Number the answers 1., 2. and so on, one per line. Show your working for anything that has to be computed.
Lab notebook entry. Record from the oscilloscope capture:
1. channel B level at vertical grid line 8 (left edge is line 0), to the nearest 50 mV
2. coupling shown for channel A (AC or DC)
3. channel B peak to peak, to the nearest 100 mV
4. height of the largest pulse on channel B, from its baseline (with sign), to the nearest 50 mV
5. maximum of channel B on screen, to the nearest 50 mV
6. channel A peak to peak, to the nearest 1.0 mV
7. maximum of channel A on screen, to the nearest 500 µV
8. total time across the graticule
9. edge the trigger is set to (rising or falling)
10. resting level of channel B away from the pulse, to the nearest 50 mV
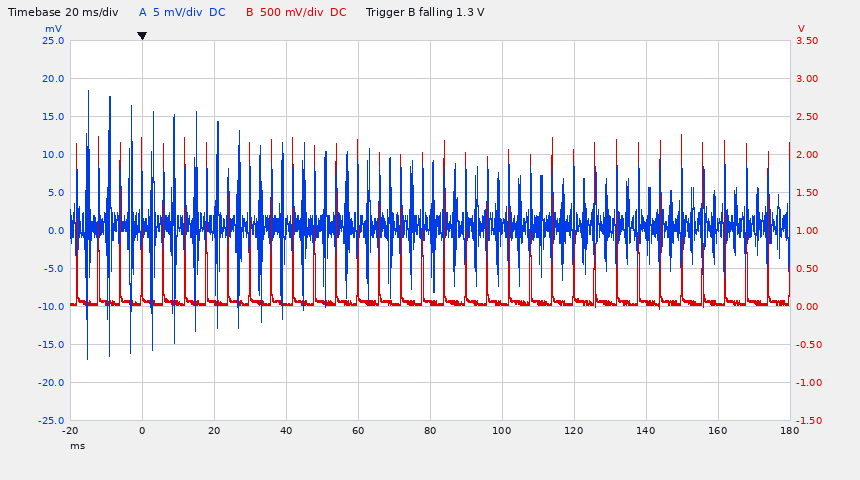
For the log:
1. 50 mV
2. DC
3. 2.30 V
4. 2.25 V − (50 mV) = +2.20 V
5. 2.25 V
6. 35.0 mV
7. 18.5 mV
8. 200 ms
9. falling
10. 50 mV
